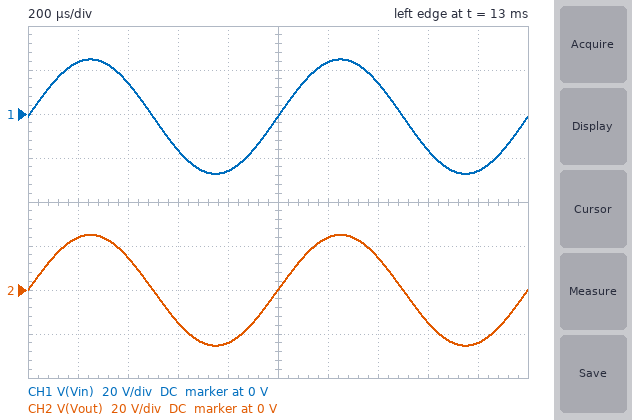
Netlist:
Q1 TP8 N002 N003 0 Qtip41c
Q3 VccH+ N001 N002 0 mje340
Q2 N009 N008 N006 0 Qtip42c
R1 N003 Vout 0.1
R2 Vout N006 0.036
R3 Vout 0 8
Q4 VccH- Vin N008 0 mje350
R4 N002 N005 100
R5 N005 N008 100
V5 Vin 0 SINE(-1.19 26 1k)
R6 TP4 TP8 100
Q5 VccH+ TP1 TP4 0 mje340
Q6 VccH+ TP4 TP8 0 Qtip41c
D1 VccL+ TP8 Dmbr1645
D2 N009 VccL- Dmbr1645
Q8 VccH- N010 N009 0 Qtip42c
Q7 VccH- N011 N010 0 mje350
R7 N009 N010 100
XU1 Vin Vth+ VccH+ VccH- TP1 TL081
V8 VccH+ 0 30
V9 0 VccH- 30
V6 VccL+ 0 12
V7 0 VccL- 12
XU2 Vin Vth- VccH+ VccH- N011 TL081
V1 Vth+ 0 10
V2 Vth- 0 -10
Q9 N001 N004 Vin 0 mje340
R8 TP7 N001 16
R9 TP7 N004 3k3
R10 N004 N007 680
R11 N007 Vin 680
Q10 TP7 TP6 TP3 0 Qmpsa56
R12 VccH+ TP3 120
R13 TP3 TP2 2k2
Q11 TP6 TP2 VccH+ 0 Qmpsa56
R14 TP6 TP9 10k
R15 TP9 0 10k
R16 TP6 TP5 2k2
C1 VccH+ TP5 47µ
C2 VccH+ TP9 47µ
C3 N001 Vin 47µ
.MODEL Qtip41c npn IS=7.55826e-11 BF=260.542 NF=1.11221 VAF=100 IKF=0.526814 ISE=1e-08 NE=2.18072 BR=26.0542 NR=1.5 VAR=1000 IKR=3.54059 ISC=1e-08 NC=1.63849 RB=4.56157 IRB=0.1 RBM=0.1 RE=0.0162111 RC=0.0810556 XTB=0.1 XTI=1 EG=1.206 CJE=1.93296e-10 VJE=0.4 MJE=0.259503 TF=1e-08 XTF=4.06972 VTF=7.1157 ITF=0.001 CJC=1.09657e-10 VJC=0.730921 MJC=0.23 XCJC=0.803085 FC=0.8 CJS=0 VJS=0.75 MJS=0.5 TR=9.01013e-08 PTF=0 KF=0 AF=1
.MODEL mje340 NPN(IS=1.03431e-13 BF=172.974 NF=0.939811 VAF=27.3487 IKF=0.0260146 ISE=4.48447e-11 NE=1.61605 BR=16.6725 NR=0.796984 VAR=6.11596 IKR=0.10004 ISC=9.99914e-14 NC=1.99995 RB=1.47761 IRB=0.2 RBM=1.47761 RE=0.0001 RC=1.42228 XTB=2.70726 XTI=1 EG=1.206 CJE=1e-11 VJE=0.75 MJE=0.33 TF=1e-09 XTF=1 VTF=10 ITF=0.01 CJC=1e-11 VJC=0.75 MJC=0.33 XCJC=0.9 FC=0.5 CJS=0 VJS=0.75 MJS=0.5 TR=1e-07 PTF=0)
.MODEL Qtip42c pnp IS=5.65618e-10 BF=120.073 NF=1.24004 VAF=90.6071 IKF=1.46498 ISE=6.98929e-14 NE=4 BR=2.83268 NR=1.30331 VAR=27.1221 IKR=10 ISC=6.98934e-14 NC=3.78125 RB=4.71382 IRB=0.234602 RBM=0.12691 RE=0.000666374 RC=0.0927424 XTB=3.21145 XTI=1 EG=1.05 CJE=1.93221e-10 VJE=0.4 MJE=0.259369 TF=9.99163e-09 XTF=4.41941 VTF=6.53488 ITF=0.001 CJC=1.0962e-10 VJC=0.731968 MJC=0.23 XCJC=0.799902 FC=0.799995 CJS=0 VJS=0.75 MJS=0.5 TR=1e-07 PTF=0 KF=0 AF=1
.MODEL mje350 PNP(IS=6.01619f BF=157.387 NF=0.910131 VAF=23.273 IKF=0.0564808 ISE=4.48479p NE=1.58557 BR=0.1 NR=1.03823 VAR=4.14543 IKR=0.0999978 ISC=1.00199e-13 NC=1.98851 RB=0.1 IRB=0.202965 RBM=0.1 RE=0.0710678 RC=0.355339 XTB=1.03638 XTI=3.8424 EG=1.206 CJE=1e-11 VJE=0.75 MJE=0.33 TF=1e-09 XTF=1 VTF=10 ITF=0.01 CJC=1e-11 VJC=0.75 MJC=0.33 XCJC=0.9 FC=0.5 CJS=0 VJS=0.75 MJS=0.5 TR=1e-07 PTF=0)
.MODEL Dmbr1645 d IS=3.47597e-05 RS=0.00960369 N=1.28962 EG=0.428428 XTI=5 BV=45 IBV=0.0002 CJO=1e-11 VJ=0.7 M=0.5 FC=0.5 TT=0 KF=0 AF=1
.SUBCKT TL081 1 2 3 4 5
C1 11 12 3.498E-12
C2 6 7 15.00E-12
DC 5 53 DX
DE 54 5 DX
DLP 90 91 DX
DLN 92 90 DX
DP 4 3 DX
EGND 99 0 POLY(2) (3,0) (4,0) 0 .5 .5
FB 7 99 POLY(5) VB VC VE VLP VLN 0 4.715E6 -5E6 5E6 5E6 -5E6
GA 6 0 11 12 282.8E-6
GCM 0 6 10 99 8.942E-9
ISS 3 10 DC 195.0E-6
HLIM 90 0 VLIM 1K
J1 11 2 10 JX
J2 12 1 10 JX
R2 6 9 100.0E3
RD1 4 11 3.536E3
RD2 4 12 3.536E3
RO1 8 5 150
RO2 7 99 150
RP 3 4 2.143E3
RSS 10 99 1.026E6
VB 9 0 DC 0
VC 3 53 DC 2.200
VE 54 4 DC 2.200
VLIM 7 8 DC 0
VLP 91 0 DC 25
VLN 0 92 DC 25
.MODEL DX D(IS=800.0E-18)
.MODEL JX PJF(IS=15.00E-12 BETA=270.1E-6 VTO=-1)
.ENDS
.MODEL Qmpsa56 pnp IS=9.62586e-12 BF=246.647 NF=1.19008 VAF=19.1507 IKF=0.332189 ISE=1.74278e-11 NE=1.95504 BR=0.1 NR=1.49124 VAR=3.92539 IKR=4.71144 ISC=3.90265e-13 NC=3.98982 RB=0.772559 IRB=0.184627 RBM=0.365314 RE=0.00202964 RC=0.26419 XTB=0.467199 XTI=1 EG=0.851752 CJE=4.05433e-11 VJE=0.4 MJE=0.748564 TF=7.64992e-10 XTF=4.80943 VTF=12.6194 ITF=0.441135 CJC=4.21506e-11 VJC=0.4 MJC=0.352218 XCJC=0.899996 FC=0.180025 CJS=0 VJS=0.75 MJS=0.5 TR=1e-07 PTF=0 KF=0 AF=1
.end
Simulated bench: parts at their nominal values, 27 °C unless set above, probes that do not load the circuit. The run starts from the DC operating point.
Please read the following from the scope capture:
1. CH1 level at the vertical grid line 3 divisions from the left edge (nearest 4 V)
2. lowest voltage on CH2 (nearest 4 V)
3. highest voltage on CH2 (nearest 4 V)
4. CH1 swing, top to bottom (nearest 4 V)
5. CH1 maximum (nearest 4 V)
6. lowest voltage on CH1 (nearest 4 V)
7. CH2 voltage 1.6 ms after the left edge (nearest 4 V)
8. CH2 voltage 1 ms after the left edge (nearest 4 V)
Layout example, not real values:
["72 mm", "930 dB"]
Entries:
["-16 V", "-24 V", "24 V", "52 V", "24 V", "-28 V", "-16 V", "0 V"]
